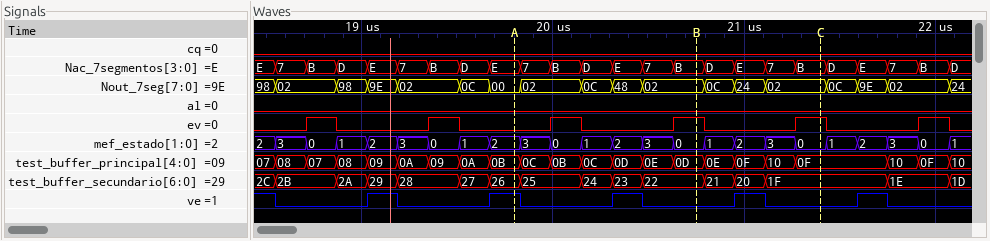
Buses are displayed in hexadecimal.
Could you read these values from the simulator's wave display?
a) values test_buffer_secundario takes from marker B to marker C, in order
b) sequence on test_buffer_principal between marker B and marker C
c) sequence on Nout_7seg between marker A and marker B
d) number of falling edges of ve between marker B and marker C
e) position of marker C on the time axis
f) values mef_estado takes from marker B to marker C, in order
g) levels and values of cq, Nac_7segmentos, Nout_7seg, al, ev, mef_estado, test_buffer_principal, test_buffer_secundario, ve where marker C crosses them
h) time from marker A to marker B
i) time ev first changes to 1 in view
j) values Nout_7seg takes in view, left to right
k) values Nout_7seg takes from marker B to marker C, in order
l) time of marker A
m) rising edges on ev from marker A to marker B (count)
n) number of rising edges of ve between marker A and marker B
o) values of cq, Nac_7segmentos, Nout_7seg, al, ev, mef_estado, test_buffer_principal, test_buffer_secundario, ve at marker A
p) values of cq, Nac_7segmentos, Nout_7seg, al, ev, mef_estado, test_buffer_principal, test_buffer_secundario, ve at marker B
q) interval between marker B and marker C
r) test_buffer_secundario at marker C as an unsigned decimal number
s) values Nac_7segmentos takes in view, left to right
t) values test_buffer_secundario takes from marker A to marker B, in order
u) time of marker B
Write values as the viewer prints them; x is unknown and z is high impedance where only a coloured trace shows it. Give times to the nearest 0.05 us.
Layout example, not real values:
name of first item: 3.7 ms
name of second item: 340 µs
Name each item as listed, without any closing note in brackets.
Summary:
values test_buffer_secundario takes from marker B to marker C, in order: 22, 21, 20, 1F
sequence on test_buffer_principal between marker B and marker C: 0D, 0E, 0F, 10, 0F
sequence on Nout_7seg between marker A and marker B: 00, 02, 0C, 48, 02
number of falling edges of ve between marker B and marker C: 1
position of marker C on the time axis: 21.4 us
values mef_estado takes from marker B to marker C, in order: 0, 1, 2, 3, 0
levels and values of cq, Nac_7segmentos, Nout_7seg, al, ev, mef_estado, test_buffer_principal, test_buffer_secundario, ve where marker C crosses them: cq=0, Nac_7segmentos=B, Nout_7seg=02, al=0, ev=1, mef_estado=0, test_buffer_principal=0F, test_buffer_secundario=1F, ve=0
time from marker A to marker B: 0.95 us
time ev first changes to 1 in view: 18.7 us
values Nout_7seg takes in view, left to right: 98, 02, 98, 9E, 02, 0C, 00, 02, 0C, 48, 02, 0C, 24, 02, 0C, 9E, 02, 24
values Nout_7seg takes from marker B to marker C, in order: 02, 0C, 24, 02
time of marker A: 19.8 us
rising edges on ev from marker A to marker B: 2
number of rising edges of ve between marker A and marker B: 1
values of cq, Nac_7segmentos, Nout_7seg, al, ev, mef_estado, test_buffer_principal, test_buffer_secundario, ve at marker A: cq=0, Nac_7segmentos=E, Nout_7seg=00, al=0, ev=0, mef_estado=2, test_buffer_principal=0B, test_buffer_secundario=26, ve=1
values of cq, Nac_7segmentos, Nout_7seg, al, ev, mef_estado, test_buffer_principal, test_buffer_secundario, ve at marker B: cq=0, Nac_7segmentos=B, Nout_7seg=02, al=0, ev=1, mef_estado=0, test_buffer_principal=0D, test_buffer_secundario=22, ve=0
interval between marker B and marker C: 0.65 us
test_buffer_secundario at marker C as an unsigned decimal number: 31
values Nac_7segmentos takes in view, left to right: E, 7, B, D, E, 7, B, D, E, 7, B, D, E, 7, B, D, E, 7, B, D, E, 7, B, D
values test_buffer_secundario takes from marker A to marker B, in order: 26, 25, 24, 23, 22
time of marker B: 20.75 us
